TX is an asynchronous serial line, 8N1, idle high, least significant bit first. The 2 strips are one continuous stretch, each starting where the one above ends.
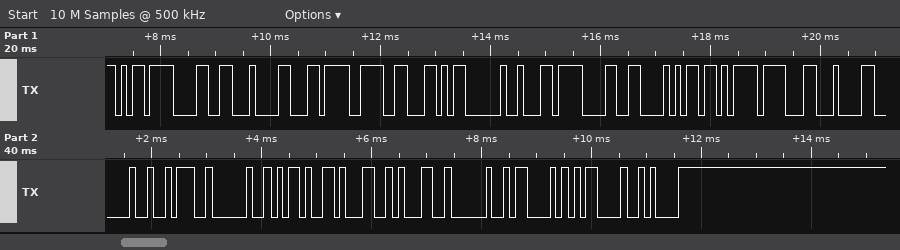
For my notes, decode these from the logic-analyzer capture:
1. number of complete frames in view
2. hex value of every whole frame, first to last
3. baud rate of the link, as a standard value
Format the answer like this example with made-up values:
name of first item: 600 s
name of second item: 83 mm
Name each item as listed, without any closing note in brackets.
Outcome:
number of complete frames in view: 23
hex value of every whole frame, first to last: ED 98 84 EC 9E AC 20 EC 98 A8 EB 8F 84 20 3A 20 2D 31 31 20 43 0D 0A
baud rate of the link, as a standard value: 9600 baud
